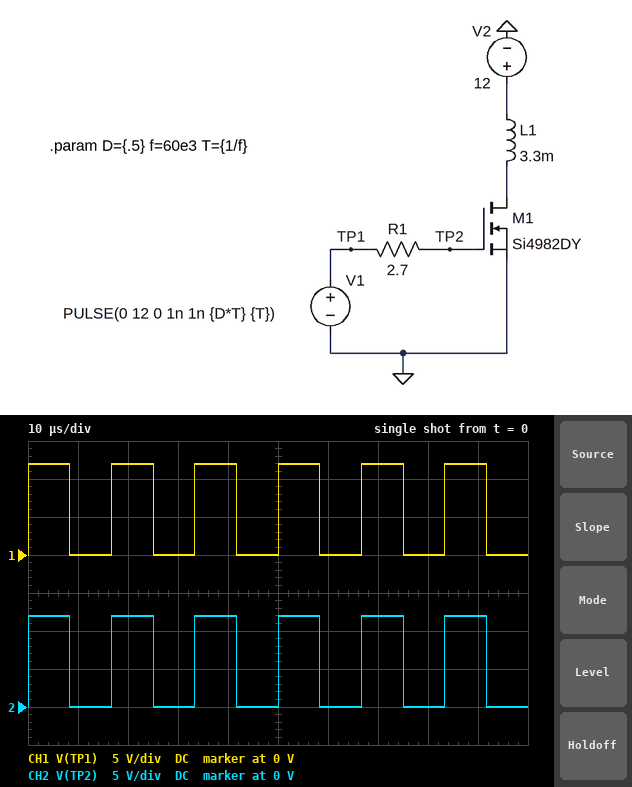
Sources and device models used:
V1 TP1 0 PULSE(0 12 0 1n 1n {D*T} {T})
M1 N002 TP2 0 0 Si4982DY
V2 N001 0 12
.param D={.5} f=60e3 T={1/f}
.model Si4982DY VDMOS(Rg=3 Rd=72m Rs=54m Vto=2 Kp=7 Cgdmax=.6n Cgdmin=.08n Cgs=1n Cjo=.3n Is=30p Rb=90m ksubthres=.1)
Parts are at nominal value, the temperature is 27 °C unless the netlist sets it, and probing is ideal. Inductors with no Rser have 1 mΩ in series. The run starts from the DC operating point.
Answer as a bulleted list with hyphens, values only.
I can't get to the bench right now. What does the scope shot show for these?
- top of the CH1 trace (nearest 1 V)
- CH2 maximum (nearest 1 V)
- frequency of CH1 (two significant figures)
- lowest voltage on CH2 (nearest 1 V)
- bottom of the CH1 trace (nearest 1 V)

- 12 V
- 12 V
- 60 kHz
- 0 V
- 0 V
